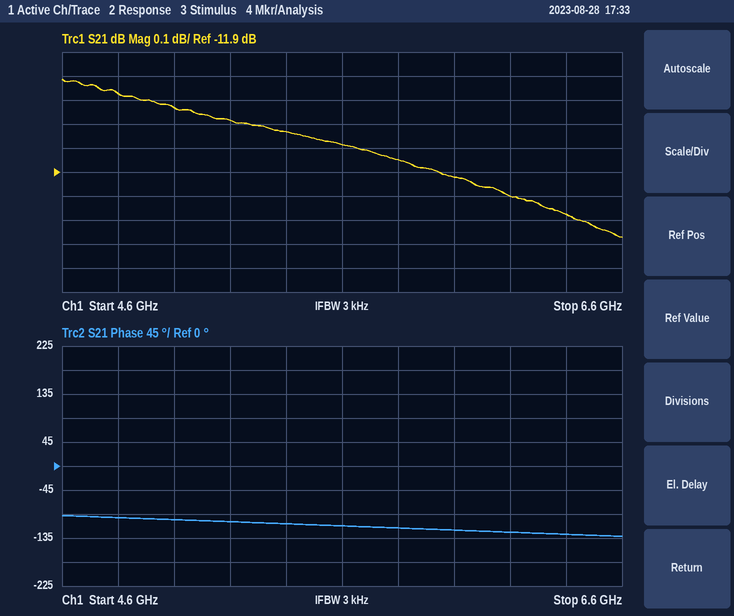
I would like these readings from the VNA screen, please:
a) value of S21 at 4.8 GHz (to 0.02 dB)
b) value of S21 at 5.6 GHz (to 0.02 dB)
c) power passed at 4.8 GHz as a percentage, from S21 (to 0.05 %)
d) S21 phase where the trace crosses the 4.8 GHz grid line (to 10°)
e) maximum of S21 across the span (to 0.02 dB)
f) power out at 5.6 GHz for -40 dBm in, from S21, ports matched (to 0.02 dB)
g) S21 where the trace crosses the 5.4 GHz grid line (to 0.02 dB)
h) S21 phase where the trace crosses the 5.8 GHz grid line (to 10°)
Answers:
-11.58 dB
-11.78 dB
6.95 %
-100°
-11.52 dB
-51.78 dBm
-11.74 dB
-120°
